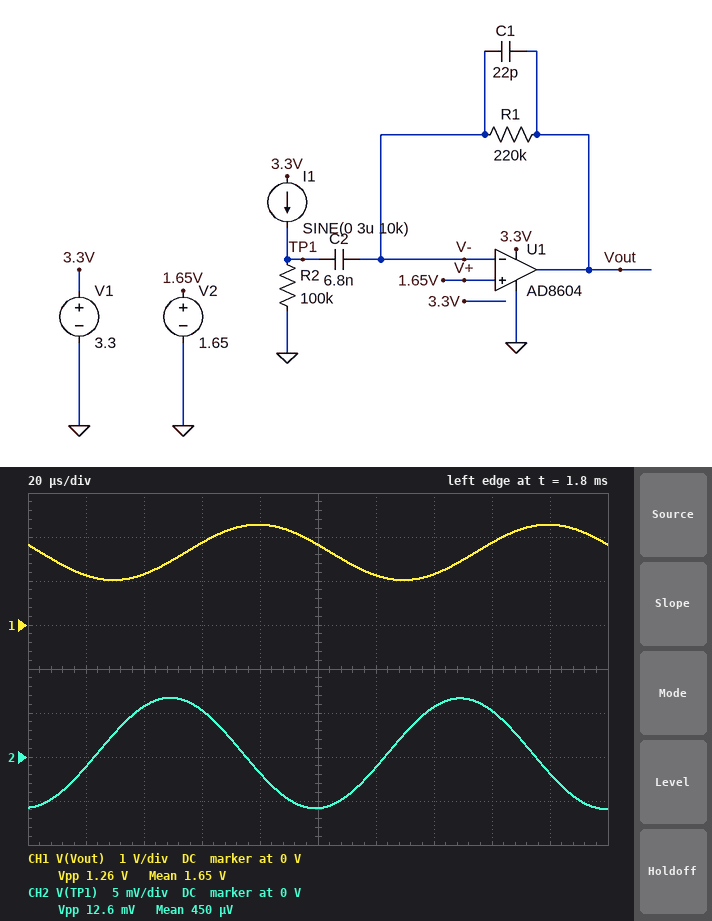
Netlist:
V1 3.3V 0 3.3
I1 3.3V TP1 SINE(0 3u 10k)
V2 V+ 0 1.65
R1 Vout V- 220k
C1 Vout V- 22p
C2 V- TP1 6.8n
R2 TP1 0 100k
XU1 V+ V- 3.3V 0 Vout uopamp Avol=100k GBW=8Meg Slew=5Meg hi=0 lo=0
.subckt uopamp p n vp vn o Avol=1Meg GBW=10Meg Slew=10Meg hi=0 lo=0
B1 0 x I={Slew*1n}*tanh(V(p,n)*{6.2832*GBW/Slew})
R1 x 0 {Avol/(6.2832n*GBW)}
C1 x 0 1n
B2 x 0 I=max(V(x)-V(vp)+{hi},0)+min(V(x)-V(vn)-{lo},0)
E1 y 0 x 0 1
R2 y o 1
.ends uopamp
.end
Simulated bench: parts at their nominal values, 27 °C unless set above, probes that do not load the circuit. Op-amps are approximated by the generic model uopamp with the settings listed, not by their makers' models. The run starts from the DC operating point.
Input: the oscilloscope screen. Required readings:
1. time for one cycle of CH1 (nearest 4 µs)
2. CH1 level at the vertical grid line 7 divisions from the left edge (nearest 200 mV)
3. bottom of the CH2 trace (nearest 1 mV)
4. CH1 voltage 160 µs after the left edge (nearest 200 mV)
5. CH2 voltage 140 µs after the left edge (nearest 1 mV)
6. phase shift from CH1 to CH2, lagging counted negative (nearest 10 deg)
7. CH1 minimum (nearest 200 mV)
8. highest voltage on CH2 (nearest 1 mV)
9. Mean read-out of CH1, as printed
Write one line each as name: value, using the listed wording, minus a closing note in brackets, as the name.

time for one cycle of CH1: 100 µs
CH1 level at the vertical grid line 7 divisions from the left edge: 1.2 V
bottom of the CH2 trace: -6 mV
CH1 voltage 160 µs after the left edge: 1.8 V
CH2 voltage 140 µs after the left edge: 6 mV
phase shift from CH1 to CH2, lagging counted negative: 110 deg
CH1 minimum: 1.0 V
highest voltage on CH2: 7 mV
Mean read-out of CH1, as printed: 1.65 V
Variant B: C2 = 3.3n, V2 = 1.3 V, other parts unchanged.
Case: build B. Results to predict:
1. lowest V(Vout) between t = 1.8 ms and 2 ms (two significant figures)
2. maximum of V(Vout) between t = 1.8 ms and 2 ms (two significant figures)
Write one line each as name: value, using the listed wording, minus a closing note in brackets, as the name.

lowest V(Vout) between t = 1.8 ms and 2 ms: 670 mV
maximum of V(Vout) between t = 1.8 ms and 2 ms: 1.9 V
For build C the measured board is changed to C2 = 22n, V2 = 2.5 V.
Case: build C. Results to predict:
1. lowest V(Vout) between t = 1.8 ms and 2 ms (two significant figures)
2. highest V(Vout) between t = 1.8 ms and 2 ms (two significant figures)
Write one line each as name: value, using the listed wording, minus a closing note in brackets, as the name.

lowest V(Vout) between t = 1.8 ms and 2 ms: 1.9 V
highest V(Vout) between t = 1.8 ms and 2 ms: 3.1 V
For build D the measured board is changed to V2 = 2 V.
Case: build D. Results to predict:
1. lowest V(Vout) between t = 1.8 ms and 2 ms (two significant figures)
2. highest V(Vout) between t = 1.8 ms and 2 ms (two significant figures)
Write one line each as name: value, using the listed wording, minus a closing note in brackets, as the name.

lowest V(Vout) between t = 1.8 ms and 2 ms: 1.4 V
highest V(Vout) between t = 1.8 ms and 2 ms: 2.6 V
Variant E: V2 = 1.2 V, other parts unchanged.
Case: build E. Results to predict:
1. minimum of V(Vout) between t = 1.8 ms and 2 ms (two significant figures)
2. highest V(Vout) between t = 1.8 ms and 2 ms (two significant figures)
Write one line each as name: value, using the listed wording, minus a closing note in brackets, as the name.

minimum of V(Vout) between t = 1.8 ms and 2 ms: 570 mV
highest V(Vout) between t = 1.8 ms and 2 ms: 1.8 V
